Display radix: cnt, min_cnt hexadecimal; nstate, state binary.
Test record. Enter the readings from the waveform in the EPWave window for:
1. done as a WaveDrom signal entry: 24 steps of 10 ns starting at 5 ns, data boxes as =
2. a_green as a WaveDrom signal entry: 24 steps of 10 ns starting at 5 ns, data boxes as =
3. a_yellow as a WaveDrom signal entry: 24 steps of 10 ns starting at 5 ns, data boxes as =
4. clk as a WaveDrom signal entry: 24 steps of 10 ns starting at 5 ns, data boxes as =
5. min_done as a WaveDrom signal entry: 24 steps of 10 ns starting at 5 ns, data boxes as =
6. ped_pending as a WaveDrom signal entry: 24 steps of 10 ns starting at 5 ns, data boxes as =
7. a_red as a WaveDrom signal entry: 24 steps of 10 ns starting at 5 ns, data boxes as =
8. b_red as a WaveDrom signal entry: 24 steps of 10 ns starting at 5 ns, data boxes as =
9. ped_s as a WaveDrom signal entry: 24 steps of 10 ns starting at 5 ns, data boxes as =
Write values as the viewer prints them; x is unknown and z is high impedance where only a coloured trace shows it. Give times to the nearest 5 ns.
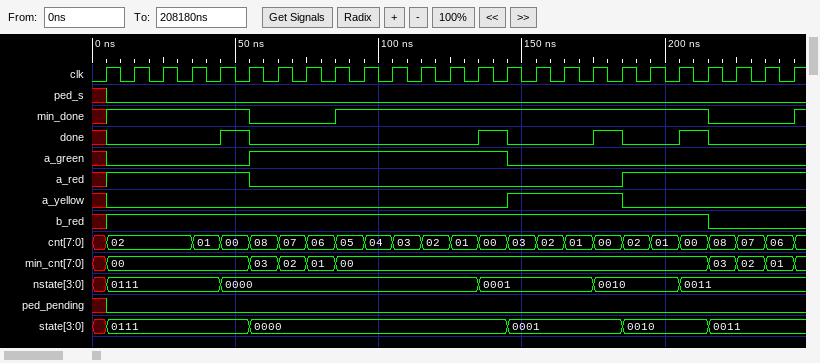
{name: 'done', wave: '0...10.......10..10.10..'}
{name: 'a_green', wave: '0....1........0.........'}
{name: 'a_yellow', wave: '0.............1...0.....'}
{name: 'clk', wave: 'p.......................'}
{name: 'min_done', wave: '1....0..1............0..'}
{name: 'ped_pending', wave: '0.......................'}
{name: 'a_red', wave: '1....0............1.....'}
{name: 'b_red', wave: '1....................0..'}
{name: 'ped_s', wave: '0.......................'}
